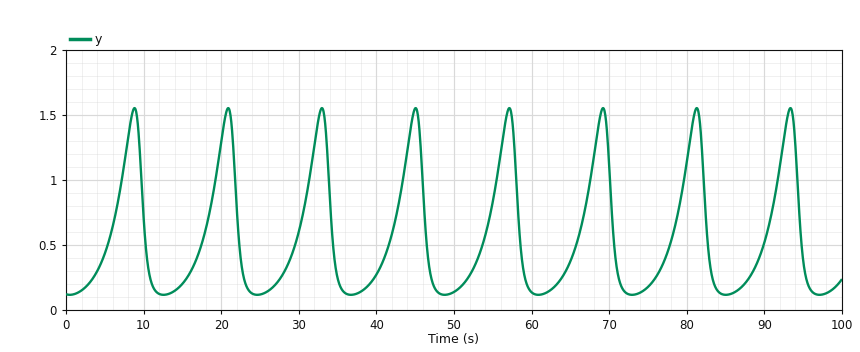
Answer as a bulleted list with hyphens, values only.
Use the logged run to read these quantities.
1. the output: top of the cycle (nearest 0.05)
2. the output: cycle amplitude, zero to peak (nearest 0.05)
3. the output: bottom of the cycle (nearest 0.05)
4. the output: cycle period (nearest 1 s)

- 1.55
- 0.70
- 0.10
- 12 s
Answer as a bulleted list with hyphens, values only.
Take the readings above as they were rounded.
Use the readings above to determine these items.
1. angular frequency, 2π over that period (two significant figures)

- 0.52 rad/s
